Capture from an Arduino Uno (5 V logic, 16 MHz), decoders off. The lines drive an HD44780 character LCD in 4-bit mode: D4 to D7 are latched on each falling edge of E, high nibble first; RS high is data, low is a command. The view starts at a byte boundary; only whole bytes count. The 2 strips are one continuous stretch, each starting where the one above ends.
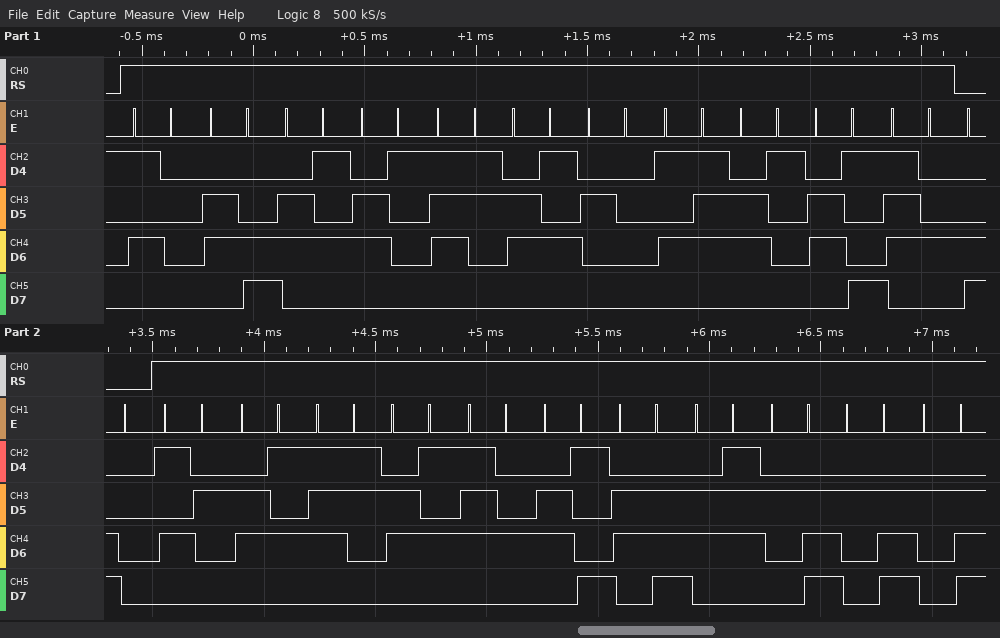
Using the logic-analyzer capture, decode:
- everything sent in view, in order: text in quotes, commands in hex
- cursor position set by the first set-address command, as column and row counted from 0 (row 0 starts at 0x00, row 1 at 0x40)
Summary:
"Please Wait" 0xC0 "Reseting..."
column 0, row 1
